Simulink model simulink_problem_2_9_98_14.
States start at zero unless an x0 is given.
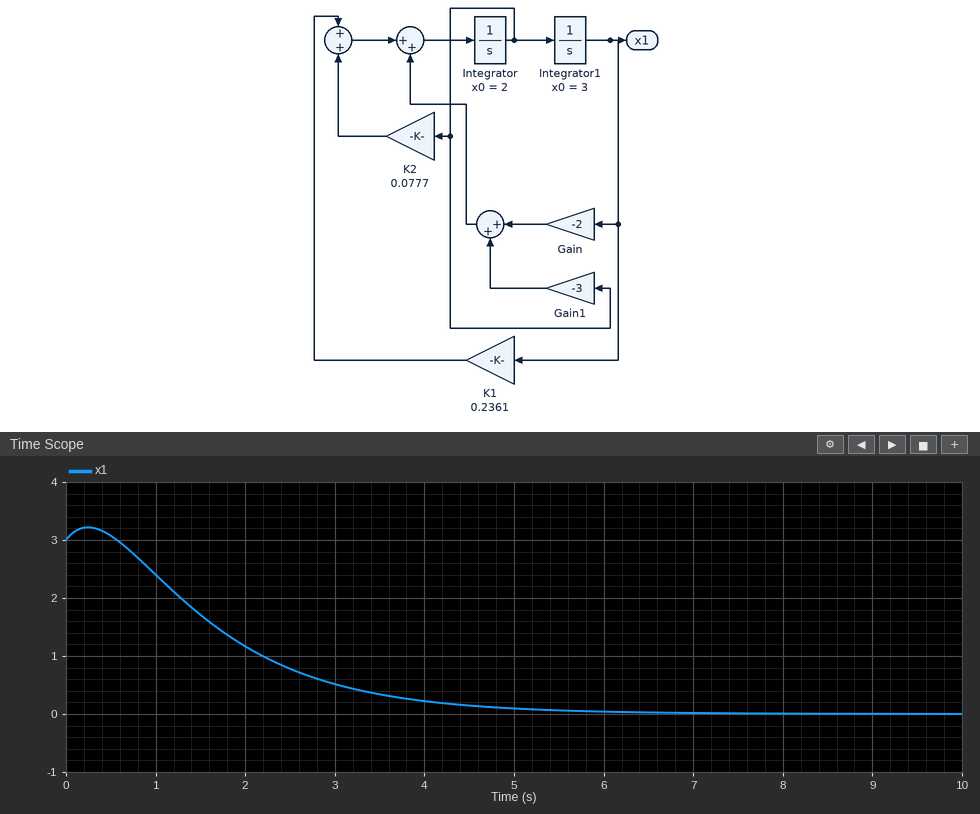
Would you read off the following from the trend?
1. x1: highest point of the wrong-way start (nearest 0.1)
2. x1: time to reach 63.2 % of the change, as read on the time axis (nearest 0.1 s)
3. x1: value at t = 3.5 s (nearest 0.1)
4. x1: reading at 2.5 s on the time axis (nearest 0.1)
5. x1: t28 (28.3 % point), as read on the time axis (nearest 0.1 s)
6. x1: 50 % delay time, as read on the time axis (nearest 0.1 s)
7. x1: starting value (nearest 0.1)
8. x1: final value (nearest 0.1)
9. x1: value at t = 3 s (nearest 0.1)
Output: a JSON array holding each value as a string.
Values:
["3.2", "2.1 s", "0.3", "0.8", "1.2 s", "1.7 s", "3.0", "0.0", "0.5"]
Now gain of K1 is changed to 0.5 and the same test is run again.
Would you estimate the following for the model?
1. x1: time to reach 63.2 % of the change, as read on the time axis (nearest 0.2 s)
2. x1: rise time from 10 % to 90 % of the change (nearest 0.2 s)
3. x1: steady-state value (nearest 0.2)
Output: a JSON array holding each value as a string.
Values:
["2.4 s", "3.4 s", "0.0"]
